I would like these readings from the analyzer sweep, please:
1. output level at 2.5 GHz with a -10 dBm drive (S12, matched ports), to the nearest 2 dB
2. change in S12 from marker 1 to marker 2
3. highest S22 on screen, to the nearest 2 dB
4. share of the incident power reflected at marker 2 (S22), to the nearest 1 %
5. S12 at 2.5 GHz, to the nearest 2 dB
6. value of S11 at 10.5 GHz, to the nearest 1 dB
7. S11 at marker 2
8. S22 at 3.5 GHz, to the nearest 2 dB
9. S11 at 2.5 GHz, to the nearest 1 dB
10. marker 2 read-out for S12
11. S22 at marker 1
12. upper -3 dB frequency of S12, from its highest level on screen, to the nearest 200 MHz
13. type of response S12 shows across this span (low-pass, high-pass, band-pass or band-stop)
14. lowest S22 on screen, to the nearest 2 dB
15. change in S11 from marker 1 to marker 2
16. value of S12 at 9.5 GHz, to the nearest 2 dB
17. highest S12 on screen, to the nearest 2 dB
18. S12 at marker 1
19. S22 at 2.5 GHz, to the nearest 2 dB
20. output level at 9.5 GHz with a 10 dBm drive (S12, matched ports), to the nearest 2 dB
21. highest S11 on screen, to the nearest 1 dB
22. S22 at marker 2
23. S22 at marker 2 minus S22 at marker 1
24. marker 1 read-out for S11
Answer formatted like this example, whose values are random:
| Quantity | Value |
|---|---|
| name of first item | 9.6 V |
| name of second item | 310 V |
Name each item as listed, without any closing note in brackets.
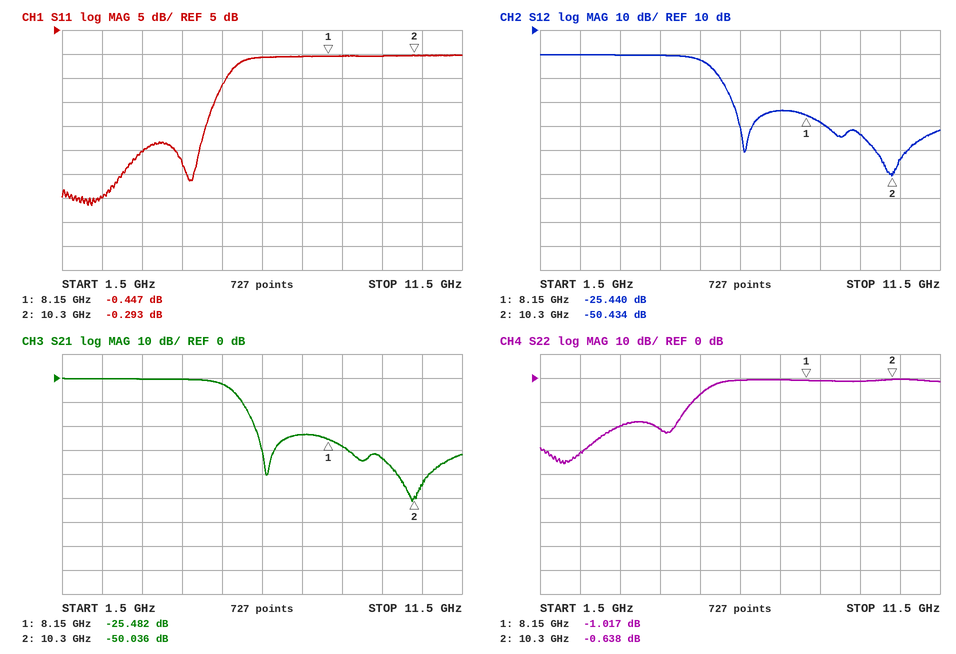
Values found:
| Quantity | Value |
|---|---|
| output level at 2.5 GHz with a -10 dBm drive (S12, matched ports), to the nearest 2 dB | -10 dBm |
| change in S12 from marker 1 to marker 2 | -24.994 dB |
| highest S22 on screen, to the nearest 2 dB | 0 dB |
| share of the incident power reflected at marker 2 (S22), to the nearest 1 % | 86 % |
| S12 at 2.5 GHz, to the nearest 2 dB | 0 dB |
| value of S11 at 10.5 GHz, to the nearest 1 dB | 0 dB |
| S11 at marker 2 | -0.293 dB |
| S22 at 3.5 GHz, to the nearest 2 dB | -20 dB |
| S11 at 2.5 GHz, to the nearest 1 dB | -30 dB |
| marker 2 read-out for S12 | -50.434 dB |
| S22 at marker 1 | -1.017 dB |
| upper -3 dB frequency of S12, from its highest level on screen, to the nearest 200 MHz | 5.6 GHz |
| type of response S12 shows across this span | low-pass |
| lowest S22 on screen, to the nearest 2 dB | -36 dB |
| change in S11 from marker 1 to marker 2 | 0.154 dB |
| value of S12 at 9.5 GHz, to the nearest 2 dB | -34 dB |
| highest S12 on screen, to the nearest 2 dB | 0 dB |
| S12 at marker 1 | -25.440 dB |
| S22 at 2.5 GHz, to the nearest 2 dB | -32 dB |
| output level at 9.5 GHz with a 10 dBm drive (S12, matched ports), to the nearest 2 dB | -24 dBm |
| highest S11 on screen, to the nearest 1 dB | 0 dB |
| S22 at marker 2 | -0.638 dB |
| S22 at marker 2 minus S22 at marker 1 | 0.379 dB |
| marker 1 read-out for S11 | -0.447 dB |
